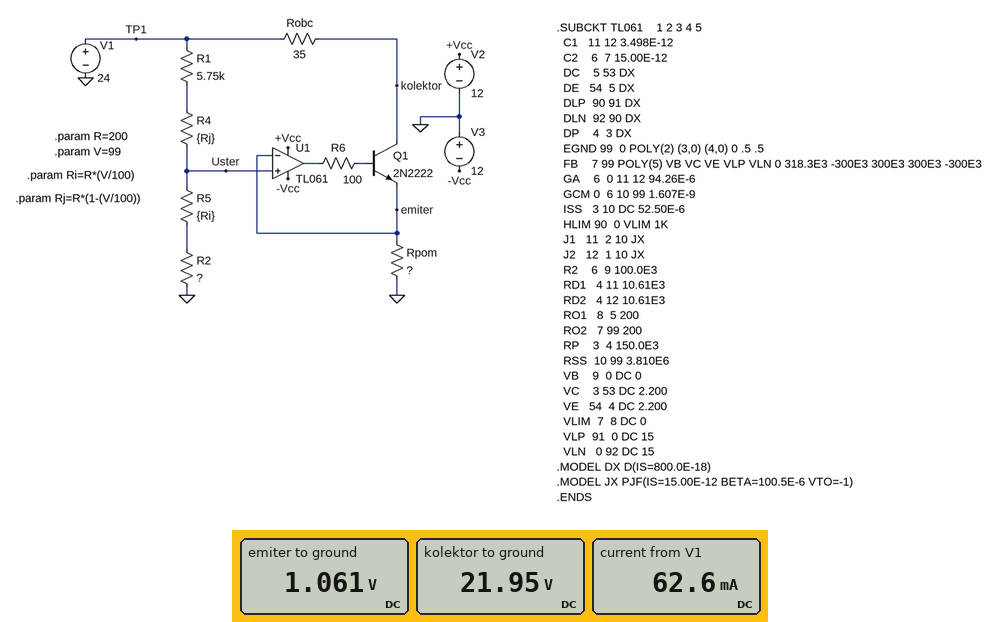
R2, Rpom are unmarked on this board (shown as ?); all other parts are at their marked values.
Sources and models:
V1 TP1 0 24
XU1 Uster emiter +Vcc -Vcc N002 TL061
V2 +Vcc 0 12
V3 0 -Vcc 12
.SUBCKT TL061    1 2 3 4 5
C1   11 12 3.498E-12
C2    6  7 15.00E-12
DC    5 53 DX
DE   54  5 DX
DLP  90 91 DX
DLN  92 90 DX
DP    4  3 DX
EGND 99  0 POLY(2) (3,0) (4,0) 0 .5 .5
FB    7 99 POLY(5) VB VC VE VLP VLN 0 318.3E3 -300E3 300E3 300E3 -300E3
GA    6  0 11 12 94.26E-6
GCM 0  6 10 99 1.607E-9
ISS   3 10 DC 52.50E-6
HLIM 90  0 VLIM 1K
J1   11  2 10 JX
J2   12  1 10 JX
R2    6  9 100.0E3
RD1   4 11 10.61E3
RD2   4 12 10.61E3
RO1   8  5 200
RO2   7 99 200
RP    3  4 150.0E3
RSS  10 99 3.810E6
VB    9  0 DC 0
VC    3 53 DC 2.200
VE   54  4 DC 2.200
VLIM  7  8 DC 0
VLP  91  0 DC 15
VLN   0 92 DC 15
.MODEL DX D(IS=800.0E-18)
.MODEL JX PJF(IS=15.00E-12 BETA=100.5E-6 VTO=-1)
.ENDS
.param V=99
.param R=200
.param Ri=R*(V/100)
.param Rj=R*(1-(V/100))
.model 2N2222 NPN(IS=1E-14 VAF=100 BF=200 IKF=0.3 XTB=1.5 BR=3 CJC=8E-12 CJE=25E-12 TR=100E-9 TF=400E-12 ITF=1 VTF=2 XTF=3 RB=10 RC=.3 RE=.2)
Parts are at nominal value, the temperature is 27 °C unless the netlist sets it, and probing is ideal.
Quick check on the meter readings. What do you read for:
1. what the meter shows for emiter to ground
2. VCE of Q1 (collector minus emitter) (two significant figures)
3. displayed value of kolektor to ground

1.061 V
21 V
21.95 V
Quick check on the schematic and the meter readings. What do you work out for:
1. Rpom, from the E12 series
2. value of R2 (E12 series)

18 Ω
68 Ω
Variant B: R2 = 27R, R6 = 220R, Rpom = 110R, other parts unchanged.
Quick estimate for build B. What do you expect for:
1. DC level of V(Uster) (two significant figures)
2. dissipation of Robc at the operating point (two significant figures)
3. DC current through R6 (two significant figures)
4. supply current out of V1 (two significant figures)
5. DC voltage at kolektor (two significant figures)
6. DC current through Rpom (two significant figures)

900 mV
2.3 mW
34 µA
12 mA
24 V
8.2 mA
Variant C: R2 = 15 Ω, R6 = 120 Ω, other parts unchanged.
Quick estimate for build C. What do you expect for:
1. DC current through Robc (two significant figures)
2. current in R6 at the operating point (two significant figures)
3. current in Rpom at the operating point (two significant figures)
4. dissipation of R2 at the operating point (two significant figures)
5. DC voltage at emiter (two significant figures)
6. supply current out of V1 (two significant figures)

47 mA
220 µA
48 mA
240 µW
860 mV
51 mA
